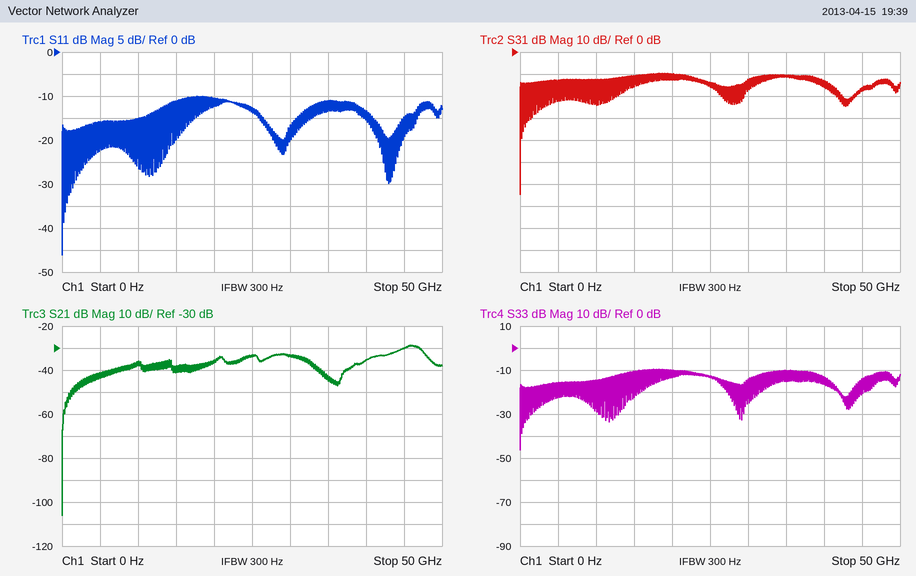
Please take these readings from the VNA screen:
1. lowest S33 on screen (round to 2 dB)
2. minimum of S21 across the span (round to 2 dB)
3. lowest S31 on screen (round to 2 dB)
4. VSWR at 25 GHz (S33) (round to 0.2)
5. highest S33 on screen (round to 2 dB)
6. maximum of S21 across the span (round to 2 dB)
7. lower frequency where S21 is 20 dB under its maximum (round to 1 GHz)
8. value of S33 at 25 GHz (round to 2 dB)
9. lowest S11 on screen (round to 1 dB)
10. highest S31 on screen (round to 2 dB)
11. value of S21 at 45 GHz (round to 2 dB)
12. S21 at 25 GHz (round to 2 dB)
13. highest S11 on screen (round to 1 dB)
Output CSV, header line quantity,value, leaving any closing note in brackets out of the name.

quantity,value
lowest S33 on screen,-46 dB
minimum of S21 across the span,-106 dB
lowest S31 on screen,-64 dB
VSWR at 25 GHz (S33),1.6
highest S33 on screen,-10 dB
maximum of S21 across the span,-28 dB
lower frequency where S21 is 20 dB under its maximum,2 GHz
value of S33 at 25 GHz,-12 dB
lowest S11 on screen,-46 dB
highest S31 on screen,-10 dB
value of S21 at 45 GHz,-30 dB
S21 at 25 GHz,-34 dB
highest S11 on screen,-10 dB
